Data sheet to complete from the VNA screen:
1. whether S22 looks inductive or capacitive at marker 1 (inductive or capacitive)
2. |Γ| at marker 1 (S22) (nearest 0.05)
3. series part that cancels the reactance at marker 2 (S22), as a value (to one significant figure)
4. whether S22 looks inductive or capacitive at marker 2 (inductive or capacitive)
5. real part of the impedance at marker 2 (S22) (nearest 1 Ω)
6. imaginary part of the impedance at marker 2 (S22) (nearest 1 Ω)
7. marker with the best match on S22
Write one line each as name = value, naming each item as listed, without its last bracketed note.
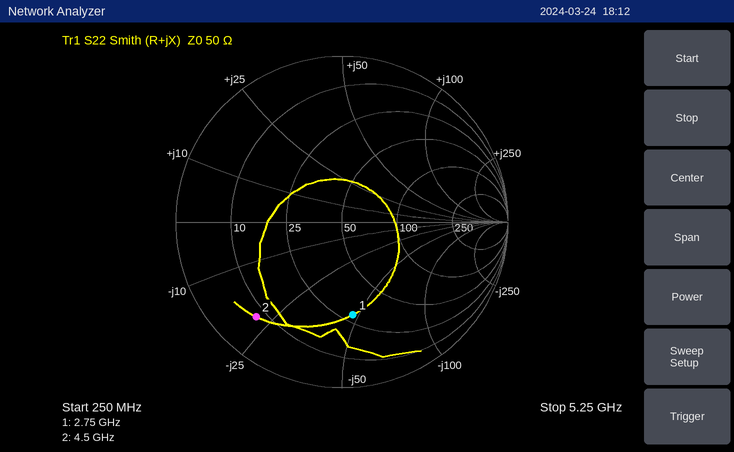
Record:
whether S22 looks inductive or capacitive at marker 1 = capacitive
|Γ| at marker 1 (S22) = 0.55
series part that cancels the reactance at marker 2 (S22), as a value = 800 pH
whether S22 looks inductive or capacitive at marker 2 = capacitive
real part of the impedance at marker 2 (S22) = 8 Ω
imaginary part of the impedance at marker 2 (S22) = -22 Ω
marker with the best match on S22 = marker 1
